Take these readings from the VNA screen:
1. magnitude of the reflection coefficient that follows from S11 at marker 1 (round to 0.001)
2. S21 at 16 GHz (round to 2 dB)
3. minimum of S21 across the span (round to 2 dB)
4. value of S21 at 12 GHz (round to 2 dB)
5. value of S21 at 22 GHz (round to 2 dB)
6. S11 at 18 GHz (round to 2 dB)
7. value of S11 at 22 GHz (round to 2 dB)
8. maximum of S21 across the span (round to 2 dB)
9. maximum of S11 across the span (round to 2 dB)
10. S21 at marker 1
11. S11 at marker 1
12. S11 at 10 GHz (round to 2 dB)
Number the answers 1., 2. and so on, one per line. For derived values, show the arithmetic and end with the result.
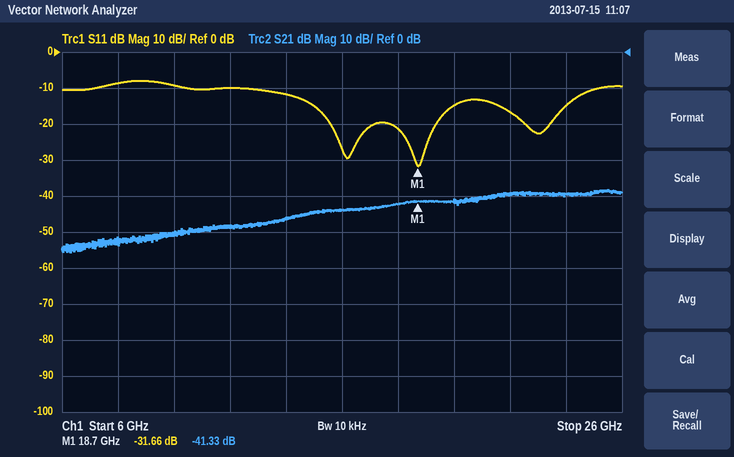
1. 10^(-31.66/20) ≈ 0.026
2. -44 dB
3. -56 dB
4. -48 dB
5. -40 dB
6. -22 dB
7. -16 dB
8. -38 dB
9. -8 dB
10. -41.33 dB
11. -31.66 dB
12. -10 dB
